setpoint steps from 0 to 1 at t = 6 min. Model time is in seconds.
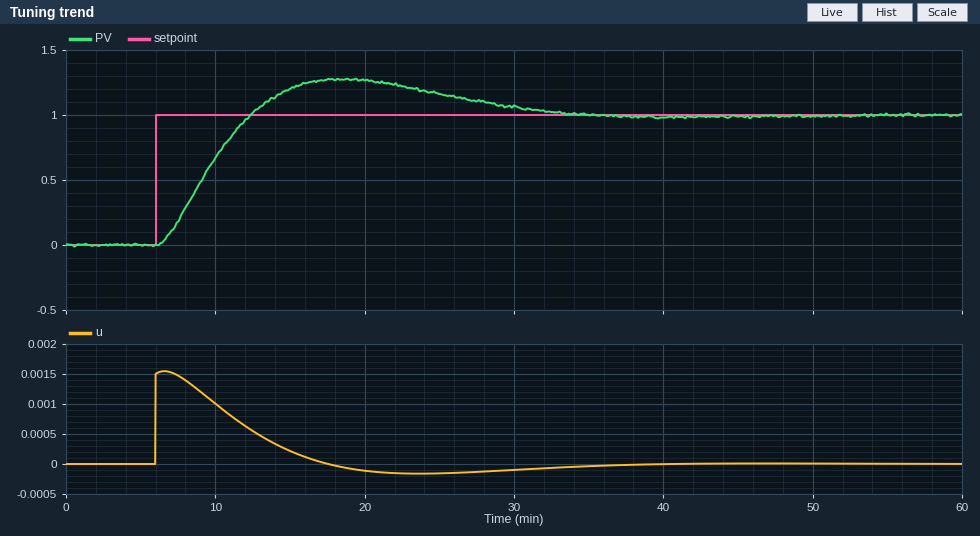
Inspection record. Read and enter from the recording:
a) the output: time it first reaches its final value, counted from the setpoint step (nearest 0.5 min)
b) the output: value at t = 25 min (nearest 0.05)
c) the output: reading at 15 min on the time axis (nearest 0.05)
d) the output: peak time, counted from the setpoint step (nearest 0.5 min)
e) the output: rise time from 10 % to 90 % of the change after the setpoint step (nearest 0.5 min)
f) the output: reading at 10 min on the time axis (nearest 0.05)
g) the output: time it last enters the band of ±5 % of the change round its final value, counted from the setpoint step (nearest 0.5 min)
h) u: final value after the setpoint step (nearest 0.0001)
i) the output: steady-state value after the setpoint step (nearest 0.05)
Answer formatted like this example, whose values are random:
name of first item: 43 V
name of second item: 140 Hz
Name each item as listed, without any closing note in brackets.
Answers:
the output: time it first reaches its final value, counted from the setpoint step: 6.5 min
the output: value at t = 25 min: 1.15
the output: reading at 15 min on the time axis: 1.20
the output: peak time, counted from the setpoint step: 12.5 min
the output: rise time from 10 % to 90 % of the change after the setpoint step: 4.5 min
the output: reading at 10 min on the time axis: 0.65
the output: time it last enters the band of ±5 % of the change round its final value, counted from the setpoint step: 24.5 min
u: final value after the setpoint step: 0.0000
the output: steady-state value after the setpoint step: 1.00
